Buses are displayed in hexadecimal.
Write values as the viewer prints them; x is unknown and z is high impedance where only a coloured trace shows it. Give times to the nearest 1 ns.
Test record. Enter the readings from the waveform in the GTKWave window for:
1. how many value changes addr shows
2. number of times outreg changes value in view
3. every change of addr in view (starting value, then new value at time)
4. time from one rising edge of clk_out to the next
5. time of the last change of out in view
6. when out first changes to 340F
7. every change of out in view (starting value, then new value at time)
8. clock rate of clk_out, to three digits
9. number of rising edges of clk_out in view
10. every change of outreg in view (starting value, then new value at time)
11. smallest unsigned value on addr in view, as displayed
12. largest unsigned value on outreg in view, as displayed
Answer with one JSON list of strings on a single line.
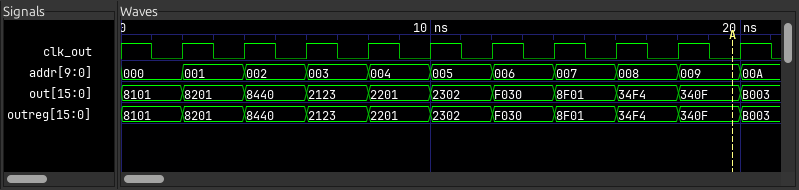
["10", "10", "000, 001 at 2 ns, 002 at 4 ns, 003 at 6 ns, 004 at 8 ns, 005 at 10 ns, 006 at 12 ns, 007 at 14 ns, 008 at 16 ns, 009 at 18 ns, 00A at 20 ns", "2 ns", "20 ns", "18 ns", "8101, 8201 at 2 ns, 8440 at 4 ns, 2123 at 6 ns, 2201 at 8 ns, 2302 at 10 ns, F030 at 12 ns, 8F01 at 14 ns, 34F4 at 16 ns, 340F at 18 ns, B003 at 20 ns", "500 MHz", "10", "8101, 8201 at 2 ns, 8440 at 4 ns, 2123 at 6 ns, 2201 at 8 ns, 2302 at 10 ns, F030 at 12 ns, 8F01 at 14 ns, 34F4 at 16 ns, 340F at 18 ns, B003 at 20 ns", "000", "F030"]
